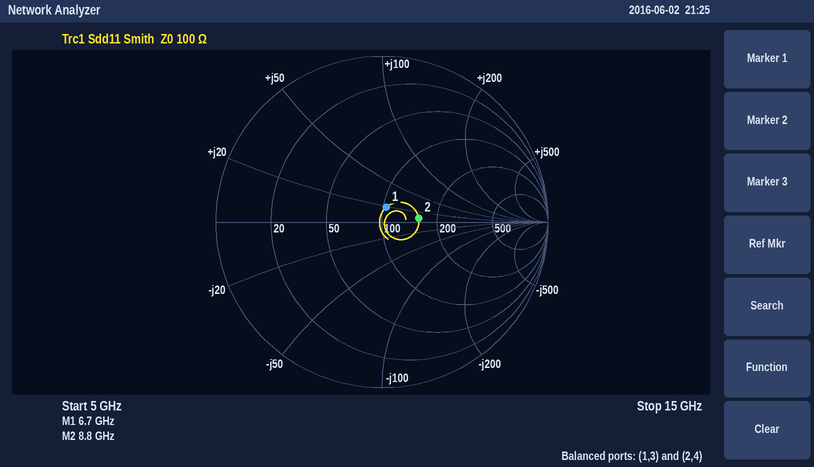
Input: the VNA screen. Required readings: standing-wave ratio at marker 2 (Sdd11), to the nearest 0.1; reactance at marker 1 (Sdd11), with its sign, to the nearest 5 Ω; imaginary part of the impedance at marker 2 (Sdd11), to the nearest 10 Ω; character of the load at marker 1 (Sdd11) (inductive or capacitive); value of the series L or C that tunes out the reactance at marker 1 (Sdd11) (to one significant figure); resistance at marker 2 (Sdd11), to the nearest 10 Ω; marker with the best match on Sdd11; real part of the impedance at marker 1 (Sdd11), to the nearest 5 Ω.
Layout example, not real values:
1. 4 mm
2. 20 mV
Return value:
1. 1.6
2. +20 Ω
3. +10 Ω
4. inductive
5. 1 pF
6. 160 Ω
7. marker 1
8. 105 Ω
